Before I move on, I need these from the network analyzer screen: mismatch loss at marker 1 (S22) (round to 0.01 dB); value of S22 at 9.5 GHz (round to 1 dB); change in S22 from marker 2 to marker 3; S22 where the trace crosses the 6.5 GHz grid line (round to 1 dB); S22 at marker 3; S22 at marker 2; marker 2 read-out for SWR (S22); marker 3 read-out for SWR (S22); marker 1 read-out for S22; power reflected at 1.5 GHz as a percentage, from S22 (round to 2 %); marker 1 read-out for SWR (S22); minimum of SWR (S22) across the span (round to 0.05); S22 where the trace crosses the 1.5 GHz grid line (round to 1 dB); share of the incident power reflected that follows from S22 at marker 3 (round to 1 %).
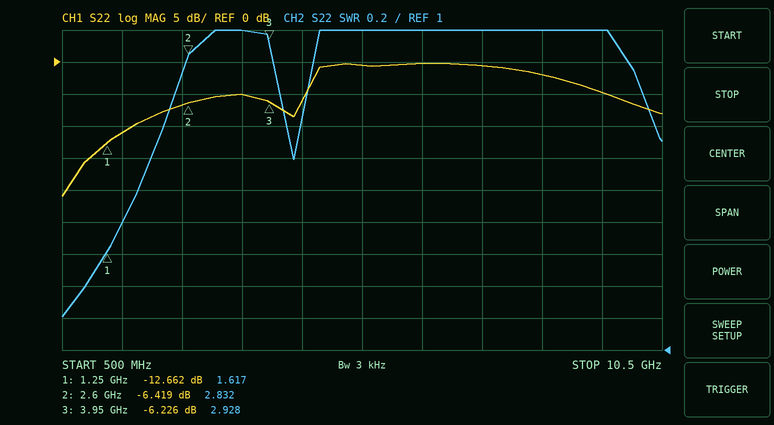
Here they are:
0.24 dB
-5 dB
0.193 dB
0 dB
-6.226 dB
-6.419 dB
2.832
2.928
-12.662 dB
8 %
1.617
1.20
-11 dB
24 %
